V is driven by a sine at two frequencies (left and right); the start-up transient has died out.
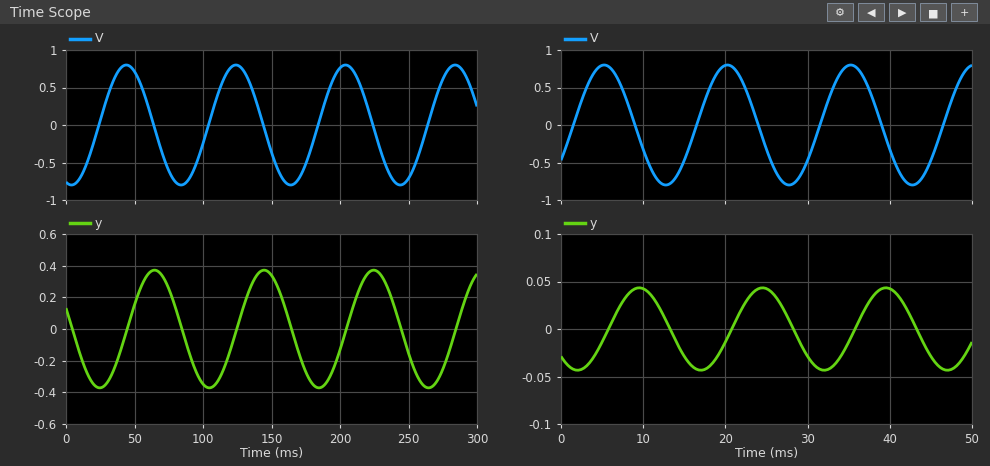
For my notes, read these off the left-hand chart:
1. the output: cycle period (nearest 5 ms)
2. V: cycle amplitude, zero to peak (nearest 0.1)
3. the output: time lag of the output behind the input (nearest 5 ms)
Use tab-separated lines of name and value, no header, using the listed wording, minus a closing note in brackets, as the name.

the output: cycle period	80 ms
V: cycle amplitude, zero to peak	0.8
the output: time lag of the output behind the input	20 ms
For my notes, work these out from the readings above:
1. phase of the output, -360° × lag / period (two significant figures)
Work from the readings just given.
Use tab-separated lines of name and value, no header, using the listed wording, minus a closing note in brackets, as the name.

phase of the output, -360° × lag / period	-90°
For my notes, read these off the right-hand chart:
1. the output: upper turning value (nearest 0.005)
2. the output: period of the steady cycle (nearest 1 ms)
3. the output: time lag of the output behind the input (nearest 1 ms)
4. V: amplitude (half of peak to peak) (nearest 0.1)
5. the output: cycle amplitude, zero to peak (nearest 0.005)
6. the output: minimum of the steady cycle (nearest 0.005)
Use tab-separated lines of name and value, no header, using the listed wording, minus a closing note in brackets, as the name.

the output: upper turning value	0.045
the output: period of the steady cycle	15 ms
the output: time lag of the output behind the input	4 ms
V: amplitude (half of peak to peak)	0.8
the output: cycle amplitude, zero to peak	0.045
the output: minimum of the steady cycle	-0.045
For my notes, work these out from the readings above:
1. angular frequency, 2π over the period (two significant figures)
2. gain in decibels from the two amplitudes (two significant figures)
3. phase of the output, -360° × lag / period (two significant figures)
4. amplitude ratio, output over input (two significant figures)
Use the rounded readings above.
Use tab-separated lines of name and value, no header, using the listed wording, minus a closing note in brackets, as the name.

angular frequency, 2π over the period	0.42 rad/ms
gain in decibels from the two amplitudes	-25 dB
phase of the output, -360° × lag / period	-96°
amplitude ratio, output over input	0.056
